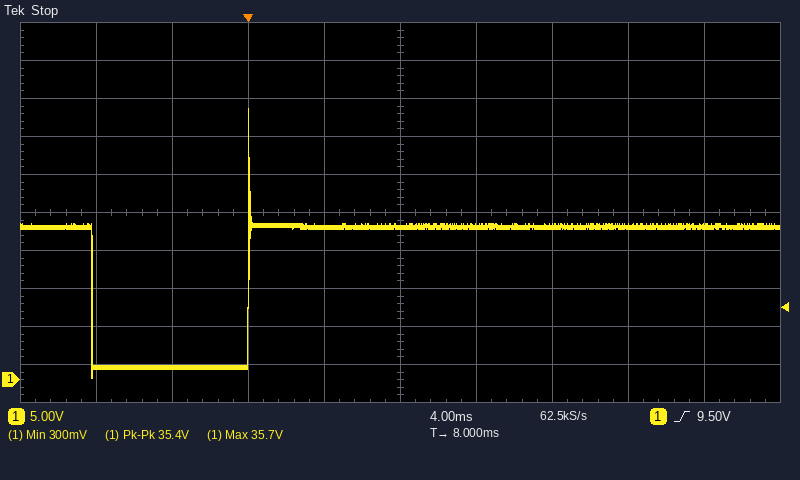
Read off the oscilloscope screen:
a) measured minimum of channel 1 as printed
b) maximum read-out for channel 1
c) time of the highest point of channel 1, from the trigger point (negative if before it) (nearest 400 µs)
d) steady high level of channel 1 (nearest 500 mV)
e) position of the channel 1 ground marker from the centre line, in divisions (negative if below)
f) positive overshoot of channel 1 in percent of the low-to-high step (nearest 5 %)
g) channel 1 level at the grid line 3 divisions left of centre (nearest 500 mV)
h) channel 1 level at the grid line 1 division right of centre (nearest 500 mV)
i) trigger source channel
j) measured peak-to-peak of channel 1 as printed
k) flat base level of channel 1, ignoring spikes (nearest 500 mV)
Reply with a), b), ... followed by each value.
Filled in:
a) 300 mV
b) 35.7 V
c) 0.0 ms
d) 20.0 V
e) -4.4 div
f) 85 %
g) 1.5 V
h) 20.0 V
i) channel 1
j) 35.4 V
k) 1.5 V
